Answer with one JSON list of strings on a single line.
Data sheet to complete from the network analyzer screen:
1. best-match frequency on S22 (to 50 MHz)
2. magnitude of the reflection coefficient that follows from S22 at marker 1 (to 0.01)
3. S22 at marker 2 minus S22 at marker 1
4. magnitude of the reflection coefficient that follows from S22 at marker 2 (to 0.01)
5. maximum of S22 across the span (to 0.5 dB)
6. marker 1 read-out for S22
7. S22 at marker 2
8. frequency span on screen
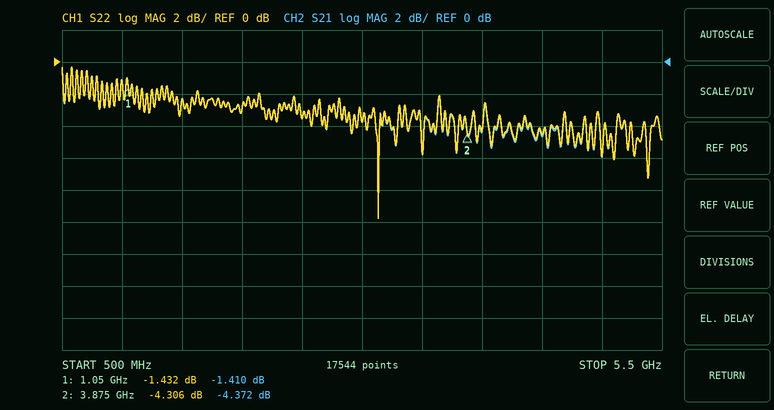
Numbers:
["3.15 GHz", "0.85", "-2.874 dB", "0.61", "-0.5 dB", "-1.432 dB", "-4.306 dB", "5 GHz"]
